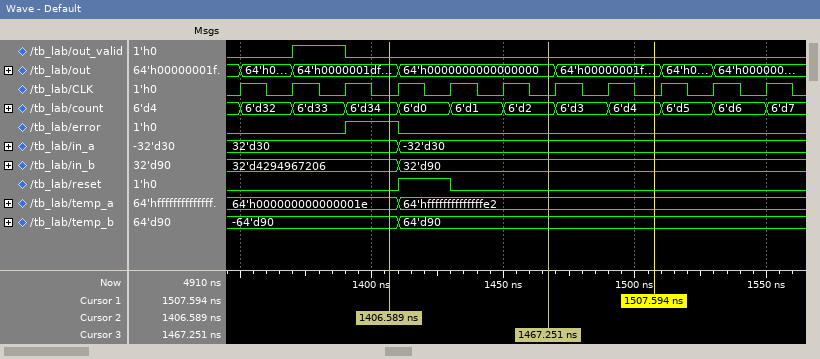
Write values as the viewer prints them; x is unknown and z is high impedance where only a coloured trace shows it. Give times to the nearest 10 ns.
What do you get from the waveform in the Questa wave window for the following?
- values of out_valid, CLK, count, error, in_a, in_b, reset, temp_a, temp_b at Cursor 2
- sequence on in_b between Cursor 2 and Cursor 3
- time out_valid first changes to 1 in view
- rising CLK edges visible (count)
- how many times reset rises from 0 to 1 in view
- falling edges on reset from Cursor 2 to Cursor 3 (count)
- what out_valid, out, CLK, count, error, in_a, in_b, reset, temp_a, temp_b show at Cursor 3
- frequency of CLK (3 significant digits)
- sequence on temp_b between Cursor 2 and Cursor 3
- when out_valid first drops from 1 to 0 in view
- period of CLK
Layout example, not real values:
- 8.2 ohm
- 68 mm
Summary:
- out_valid=0, CLK=0, count=6'd34, error=1, in_a=32'd30, in_b=32'd4294967206, reset=0, temp_a=64'h000000000000001e, temp_b=-64'd90
- 32'd4294967206, 32'd90
- 1370 ns
- 11
- 1
- 1
- out_valid=0, out=64'h0000000000000000, CLK=0, count=6'd2, error=0, in_a=-32'd30, in_b=32'd90, reset=0, temp_a=64'hffffffffffffffe2, temp_b=64'd90
- 50.0 MHz
- -64'd90, 64'd90
- 1390 ns
- 20 ns
